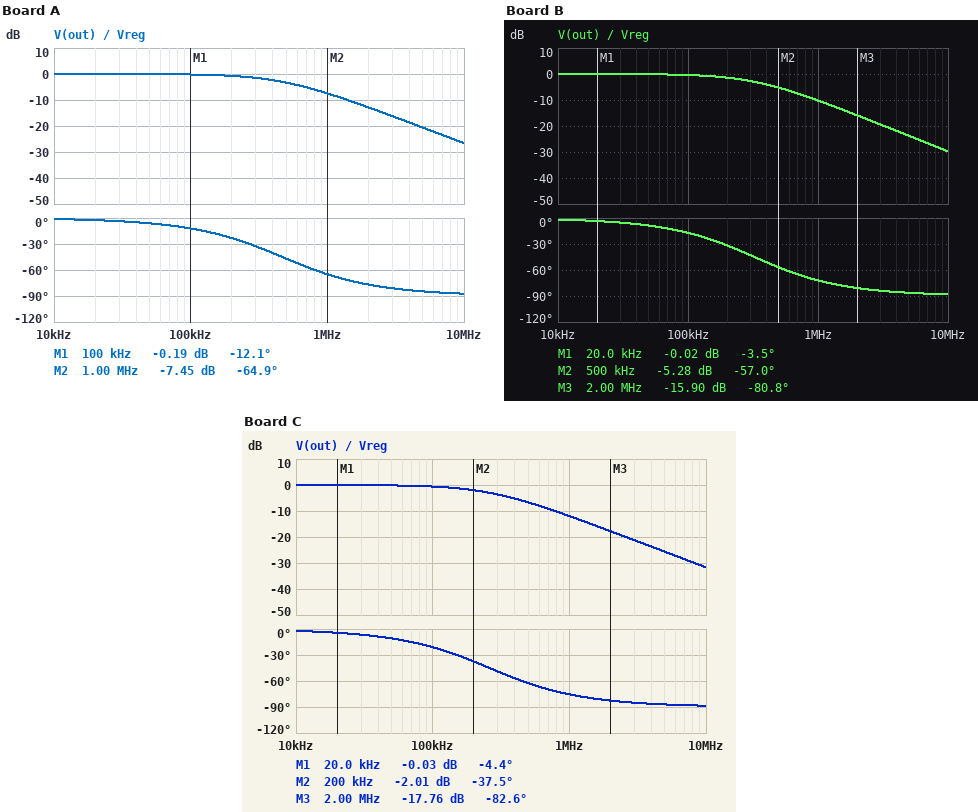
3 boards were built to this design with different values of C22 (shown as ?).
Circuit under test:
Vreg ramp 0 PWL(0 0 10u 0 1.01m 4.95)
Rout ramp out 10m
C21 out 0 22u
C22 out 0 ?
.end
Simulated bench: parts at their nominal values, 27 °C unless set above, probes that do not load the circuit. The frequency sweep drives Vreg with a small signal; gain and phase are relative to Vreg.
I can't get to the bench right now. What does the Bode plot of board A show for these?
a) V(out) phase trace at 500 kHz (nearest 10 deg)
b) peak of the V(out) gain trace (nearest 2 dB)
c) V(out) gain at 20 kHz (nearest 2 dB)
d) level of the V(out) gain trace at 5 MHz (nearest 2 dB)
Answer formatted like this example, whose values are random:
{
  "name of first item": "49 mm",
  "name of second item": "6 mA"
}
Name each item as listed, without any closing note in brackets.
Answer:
{
  "V(out) phase trace at 500 kHz": "-50 deg",
  "peak of the V(out) gain trace": "0 dB",
  "V(out) gain at 20 kHz": "0 dB",
  "level of the V(out) gain trace at 5 MHz": "-20 dB"
}
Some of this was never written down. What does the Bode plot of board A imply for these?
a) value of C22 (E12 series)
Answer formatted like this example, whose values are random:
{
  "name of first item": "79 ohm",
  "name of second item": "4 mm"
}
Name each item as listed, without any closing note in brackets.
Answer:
{
  "value of C22": "12 µF"
}
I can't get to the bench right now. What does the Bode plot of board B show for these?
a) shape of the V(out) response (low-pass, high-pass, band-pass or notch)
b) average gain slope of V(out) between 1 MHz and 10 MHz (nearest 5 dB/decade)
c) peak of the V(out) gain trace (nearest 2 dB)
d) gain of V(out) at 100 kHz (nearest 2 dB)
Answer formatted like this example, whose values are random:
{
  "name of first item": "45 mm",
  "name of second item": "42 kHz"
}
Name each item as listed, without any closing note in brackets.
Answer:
{
  "shape of the V(out) response": "low-pass",
  "average gain slope of V(out) between 1 MHz and 10 MHz": "-20 dB/decade",
  "peak of the V(out) gain trace": "0 dB",
  "gain of V(out) at 100 kHz": "0 dB"
}
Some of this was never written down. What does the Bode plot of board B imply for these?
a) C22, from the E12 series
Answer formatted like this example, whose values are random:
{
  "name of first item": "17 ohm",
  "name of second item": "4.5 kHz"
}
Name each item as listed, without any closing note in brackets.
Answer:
{
  "C22, from the E12 series": "27 µF"
}
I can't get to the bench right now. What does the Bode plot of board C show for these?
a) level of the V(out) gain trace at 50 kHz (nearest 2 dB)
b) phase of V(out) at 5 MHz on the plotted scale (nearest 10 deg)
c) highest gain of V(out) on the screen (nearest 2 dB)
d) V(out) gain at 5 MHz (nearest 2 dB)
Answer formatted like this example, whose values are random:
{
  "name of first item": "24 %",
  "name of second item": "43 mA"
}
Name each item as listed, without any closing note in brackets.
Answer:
{
  "level of the V(out) gain trace at 50 kHz": "0 dB",
  "phase of V(out) at 5 MHz on the plotted scale": "-90 deg",
  "highest gain of V(out) on the screen": "0 dB",
  "V(out) gain at 5 MHz": "-26 dB"
}
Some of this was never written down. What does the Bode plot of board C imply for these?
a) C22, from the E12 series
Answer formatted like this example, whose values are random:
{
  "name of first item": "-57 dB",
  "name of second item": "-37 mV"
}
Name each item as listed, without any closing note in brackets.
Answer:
{
  "C22, from the E12 series": "39 µF"
}
